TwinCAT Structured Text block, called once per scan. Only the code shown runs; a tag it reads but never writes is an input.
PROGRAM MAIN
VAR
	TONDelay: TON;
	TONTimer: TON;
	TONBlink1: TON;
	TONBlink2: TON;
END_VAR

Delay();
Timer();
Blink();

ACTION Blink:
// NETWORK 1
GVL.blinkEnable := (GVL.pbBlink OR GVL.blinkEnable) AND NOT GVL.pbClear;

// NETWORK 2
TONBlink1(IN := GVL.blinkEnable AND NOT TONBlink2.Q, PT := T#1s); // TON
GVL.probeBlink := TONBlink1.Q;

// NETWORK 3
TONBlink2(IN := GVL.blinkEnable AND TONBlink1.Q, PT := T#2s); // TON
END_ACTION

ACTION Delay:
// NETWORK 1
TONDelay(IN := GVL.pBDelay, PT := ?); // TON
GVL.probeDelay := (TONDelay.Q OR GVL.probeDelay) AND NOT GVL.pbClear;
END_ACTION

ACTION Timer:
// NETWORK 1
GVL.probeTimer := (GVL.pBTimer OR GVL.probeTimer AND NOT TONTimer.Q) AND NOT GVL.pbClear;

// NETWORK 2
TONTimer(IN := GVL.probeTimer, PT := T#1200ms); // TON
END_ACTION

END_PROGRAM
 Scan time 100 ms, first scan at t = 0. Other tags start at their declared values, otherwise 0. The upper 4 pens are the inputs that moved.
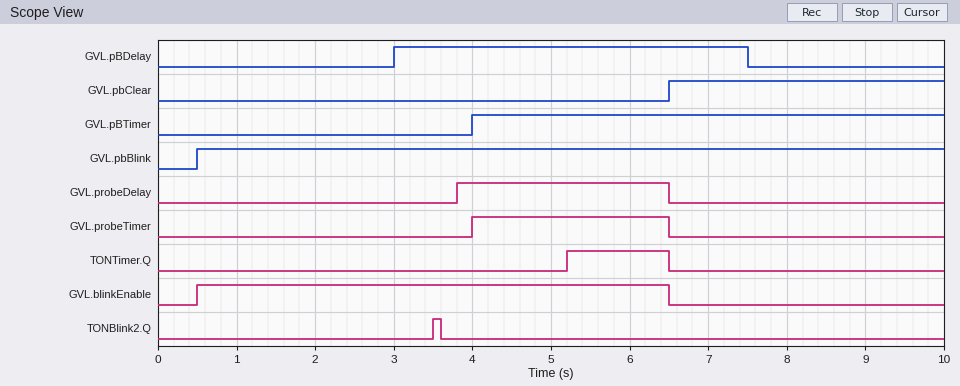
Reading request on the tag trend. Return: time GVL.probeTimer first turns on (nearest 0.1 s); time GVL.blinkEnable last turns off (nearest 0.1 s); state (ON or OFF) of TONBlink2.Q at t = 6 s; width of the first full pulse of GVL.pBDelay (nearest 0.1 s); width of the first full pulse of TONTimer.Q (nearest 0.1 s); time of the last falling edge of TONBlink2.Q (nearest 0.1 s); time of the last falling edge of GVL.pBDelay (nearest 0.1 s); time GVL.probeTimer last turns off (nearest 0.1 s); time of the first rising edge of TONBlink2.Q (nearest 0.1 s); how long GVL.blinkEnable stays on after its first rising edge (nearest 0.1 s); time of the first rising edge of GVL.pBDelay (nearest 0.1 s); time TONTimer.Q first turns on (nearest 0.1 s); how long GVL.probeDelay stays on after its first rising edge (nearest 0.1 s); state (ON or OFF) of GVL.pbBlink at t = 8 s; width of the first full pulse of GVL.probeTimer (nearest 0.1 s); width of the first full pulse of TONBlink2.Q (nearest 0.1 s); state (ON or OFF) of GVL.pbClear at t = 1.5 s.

4.0 s
6.5 s
OFF
4.5 s
1.3 s
3.6 s
7.5 s
6.5 s
3.5 s
6.0 s
3.0 s
5.2 s
2.7 s
ON
2.5 s
0.1 s
OFF
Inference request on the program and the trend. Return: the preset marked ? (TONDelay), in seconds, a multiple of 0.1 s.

0.8 s
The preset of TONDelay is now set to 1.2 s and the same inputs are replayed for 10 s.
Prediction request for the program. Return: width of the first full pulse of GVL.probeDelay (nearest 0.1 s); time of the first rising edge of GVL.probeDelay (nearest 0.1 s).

2.3 s
4.2 s
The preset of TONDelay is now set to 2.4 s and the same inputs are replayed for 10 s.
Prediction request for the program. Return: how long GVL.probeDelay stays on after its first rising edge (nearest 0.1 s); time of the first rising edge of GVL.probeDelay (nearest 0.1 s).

1.1 s
5.4 s
